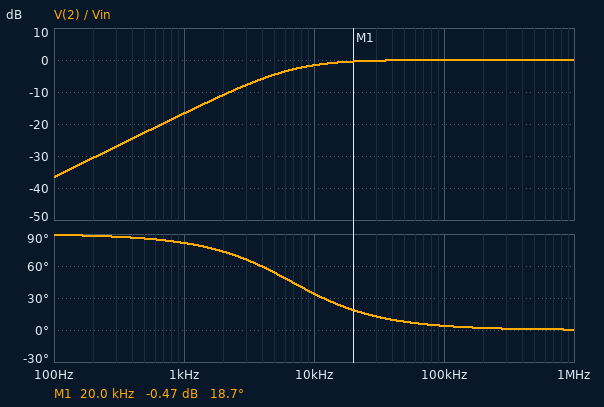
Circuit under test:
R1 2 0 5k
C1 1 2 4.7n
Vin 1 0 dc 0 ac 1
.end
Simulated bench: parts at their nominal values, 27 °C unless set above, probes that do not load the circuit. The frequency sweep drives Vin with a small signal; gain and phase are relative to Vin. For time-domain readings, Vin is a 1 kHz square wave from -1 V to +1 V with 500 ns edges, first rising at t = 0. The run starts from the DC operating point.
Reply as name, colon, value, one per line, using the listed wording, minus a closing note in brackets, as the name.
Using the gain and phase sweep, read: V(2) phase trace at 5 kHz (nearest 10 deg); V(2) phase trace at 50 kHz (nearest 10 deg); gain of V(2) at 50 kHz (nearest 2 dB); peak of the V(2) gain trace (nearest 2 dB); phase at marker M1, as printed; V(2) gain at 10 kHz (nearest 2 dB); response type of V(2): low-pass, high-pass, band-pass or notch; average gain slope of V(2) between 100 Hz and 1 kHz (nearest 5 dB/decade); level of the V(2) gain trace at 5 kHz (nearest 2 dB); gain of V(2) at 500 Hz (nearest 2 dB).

V(2) phase trace at 5 kHz: 50 deg
V(2) phase trace at 50 kHz: 10 deg
gain of V(2) at 50 kHz: 0 dB
peak of the V(2) gain trace: 0 dB
phase at marker M1, as printed: 18.7 deg
V(2) gain at 10 kHz: -2 dB
response type of V(2): low-pass, high-pass, band-pass or notch: high-pass
average gain slope of V(2) between 100 Hz and 1 kHz: 20 dB/decade
level of the V(2) gain trace at 5 kHz: -4 dB
gain of V(2) at 500 Hz: -22 dB
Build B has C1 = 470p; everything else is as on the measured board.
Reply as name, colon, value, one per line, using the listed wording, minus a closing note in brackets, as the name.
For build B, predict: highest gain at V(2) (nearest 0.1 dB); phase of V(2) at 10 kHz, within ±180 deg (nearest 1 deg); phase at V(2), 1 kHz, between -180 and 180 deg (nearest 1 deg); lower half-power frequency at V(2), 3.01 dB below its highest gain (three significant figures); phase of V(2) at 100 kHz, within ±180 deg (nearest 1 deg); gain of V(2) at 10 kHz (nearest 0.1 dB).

highest gain at V(2): 0 dB
phase of V(2) at 10 kHz, within ±180 deg: 82 deg
phase at V(2), 1 kHz, between -180 and 180 deg: 89 deg
lower half-power frequency at V(2), 3.01 dB below its highest gain: 67.7 kHz
phase of V(2) at 100 kHz, within ±180 deg: 34 deg
gain of V(2) at 10 kHz: -16.7 dB
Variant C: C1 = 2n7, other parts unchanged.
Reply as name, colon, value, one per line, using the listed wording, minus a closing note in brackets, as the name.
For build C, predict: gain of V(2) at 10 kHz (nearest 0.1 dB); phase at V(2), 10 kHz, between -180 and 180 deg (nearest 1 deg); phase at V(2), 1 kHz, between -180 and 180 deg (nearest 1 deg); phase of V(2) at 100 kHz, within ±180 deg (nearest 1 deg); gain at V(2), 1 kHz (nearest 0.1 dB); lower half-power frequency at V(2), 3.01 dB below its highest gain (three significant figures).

gain of V(2) at 10 kHz: -3.8 dB
phase at V(2), 10 kHz, between -180 and 180 deg: 50 deg
phase at V(2), 1 kHz, between -180 and 180 deg: 85 deg
phase of V(2) at 100 kHz, within ±180 deg: 7 deg
gain at V(2), 1 kHz: -21.5 dB
lower half-power frequency at V(2), 3.01 dB below its highest gain: 11.8 kHz
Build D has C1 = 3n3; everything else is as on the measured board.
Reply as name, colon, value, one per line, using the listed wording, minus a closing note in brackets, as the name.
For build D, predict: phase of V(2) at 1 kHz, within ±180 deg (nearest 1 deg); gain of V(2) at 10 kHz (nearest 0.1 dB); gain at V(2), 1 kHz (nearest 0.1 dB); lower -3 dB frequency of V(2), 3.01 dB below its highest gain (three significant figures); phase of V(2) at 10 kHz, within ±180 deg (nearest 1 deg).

phase of V(2) at 1 kHz, within ±180 deg: 84 deg
gain of V(2) at 10 kHz: -2.9 dB
gain at V(2), 1 kHz: -19.7 dB
lower -3 dB frequency of V(2), 3.01 dB below its highest gain: 9.65 kHz
phase of V(2) at 10 kHz, within ±180 deg: 44 deg
